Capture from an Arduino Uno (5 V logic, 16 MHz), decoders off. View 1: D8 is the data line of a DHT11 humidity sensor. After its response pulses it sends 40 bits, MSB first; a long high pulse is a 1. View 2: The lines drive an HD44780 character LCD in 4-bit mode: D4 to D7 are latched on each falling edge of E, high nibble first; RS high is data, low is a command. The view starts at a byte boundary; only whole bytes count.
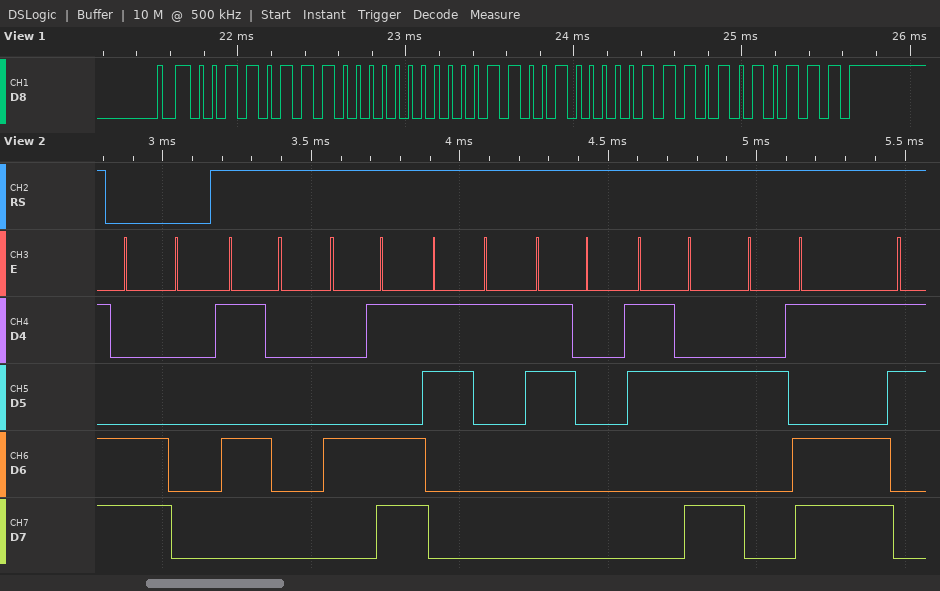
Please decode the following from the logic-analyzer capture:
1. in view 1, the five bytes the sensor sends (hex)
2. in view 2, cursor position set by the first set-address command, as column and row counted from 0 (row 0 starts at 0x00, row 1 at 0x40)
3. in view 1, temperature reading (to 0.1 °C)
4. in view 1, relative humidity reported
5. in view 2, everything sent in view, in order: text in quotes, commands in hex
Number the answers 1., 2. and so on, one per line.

1. 37 00 19 07 57
2. column 0, row 1
3. 25.7 °C
4. 55 %
5. 0xC0 "PM10:-"
